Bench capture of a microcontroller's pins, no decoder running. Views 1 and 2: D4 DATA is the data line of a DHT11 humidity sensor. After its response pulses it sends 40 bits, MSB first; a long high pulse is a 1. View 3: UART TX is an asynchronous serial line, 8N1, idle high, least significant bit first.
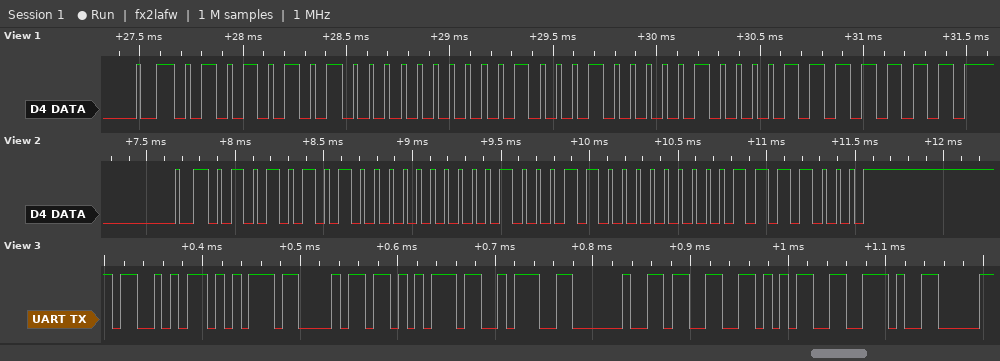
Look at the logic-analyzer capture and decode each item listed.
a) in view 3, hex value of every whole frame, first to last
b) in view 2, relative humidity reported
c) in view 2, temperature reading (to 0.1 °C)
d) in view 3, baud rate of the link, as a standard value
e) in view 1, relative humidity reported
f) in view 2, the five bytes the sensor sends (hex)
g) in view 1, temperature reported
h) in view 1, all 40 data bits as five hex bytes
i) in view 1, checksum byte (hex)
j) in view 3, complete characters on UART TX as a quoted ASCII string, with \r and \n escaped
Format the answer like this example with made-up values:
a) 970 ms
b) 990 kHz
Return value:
a) 0x53 0x75 0x68 0x75 0x3A 0x20 0x33 0x35 0x2E
b) 85 %
c) 35.0 °C
d) 115200 baud
e) 85 %
f) 55 00 23 00 78
g) 34.8 °C
h) 55 00 22 08 7F
i) 0x7F
j) "Suhu: 35."
